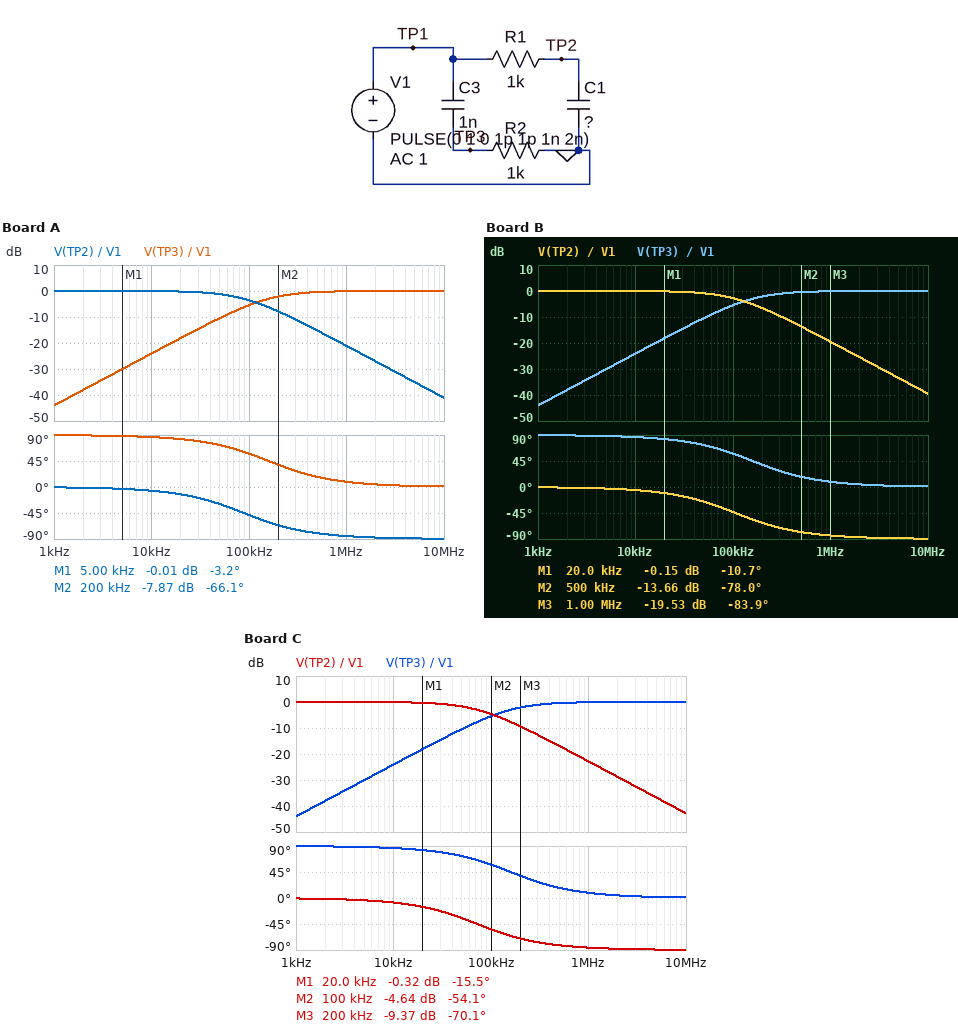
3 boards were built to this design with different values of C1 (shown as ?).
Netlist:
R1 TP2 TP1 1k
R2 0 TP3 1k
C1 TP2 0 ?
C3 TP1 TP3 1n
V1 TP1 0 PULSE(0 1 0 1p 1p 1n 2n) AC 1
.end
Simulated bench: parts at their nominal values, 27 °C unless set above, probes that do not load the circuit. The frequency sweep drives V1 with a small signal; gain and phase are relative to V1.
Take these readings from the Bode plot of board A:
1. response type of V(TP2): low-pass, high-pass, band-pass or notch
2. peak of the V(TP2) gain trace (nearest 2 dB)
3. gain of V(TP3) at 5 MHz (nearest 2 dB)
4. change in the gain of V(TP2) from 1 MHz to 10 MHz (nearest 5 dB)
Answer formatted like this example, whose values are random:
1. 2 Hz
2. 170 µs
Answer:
1. low-pass
2. 0 dB
3. 0 dB
4. -20 dB
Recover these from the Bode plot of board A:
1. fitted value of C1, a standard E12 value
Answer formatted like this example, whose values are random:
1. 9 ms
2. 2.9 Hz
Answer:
1. 1.8 nF
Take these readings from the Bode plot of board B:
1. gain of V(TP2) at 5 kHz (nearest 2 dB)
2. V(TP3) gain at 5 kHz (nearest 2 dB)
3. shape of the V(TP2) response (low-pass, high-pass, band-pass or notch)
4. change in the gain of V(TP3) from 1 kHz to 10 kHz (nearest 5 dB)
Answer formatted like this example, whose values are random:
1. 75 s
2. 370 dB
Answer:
1. 0 dB
2. -30 dB
3. low-pass
4. 20 dB
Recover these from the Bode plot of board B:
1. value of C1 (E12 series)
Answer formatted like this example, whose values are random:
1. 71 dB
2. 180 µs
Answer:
1. 1.5 nF
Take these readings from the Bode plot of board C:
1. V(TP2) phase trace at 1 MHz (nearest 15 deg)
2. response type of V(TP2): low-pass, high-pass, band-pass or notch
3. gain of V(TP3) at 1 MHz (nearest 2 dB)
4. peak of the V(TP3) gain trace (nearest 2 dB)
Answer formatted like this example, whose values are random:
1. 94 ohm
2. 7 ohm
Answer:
1. -90 deg
2. low-pass
3. 0 dB
4. 0 dB
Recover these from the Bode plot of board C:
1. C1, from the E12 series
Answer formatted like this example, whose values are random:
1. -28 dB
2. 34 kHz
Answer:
1. 2.2 nF
